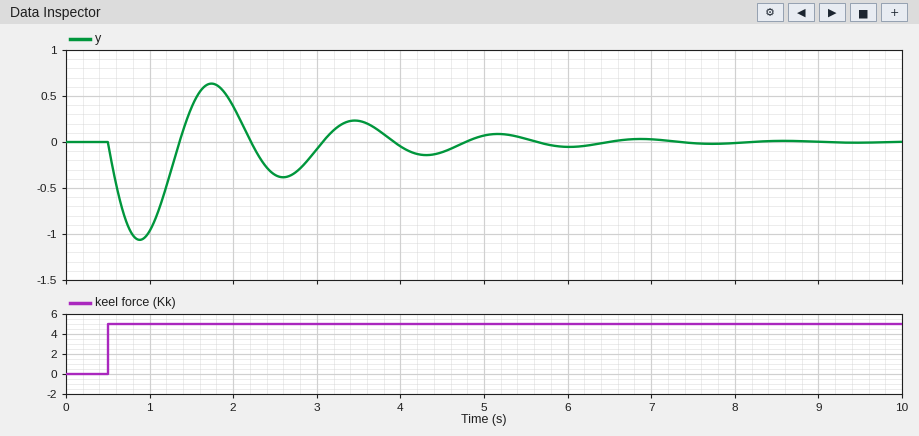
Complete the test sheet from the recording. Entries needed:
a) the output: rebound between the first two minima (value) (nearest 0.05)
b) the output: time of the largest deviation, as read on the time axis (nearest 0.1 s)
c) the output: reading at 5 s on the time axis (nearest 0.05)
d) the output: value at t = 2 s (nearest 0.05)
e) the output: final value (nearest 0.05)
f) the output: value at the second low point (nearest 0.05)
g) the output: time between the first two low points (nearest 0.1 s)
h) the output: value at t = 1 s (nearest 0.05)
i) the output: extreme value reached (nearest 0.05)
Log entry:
0.65
0.9 s
0.05
0.40
0.00
-0.40
1.7 s
-0.95
-1.05
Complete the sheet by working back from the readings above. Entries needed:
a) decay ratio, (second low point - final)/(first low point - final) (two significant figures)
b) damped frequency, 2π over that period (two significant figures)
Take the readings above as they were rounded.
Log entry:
0.38
3.7 rad/s
